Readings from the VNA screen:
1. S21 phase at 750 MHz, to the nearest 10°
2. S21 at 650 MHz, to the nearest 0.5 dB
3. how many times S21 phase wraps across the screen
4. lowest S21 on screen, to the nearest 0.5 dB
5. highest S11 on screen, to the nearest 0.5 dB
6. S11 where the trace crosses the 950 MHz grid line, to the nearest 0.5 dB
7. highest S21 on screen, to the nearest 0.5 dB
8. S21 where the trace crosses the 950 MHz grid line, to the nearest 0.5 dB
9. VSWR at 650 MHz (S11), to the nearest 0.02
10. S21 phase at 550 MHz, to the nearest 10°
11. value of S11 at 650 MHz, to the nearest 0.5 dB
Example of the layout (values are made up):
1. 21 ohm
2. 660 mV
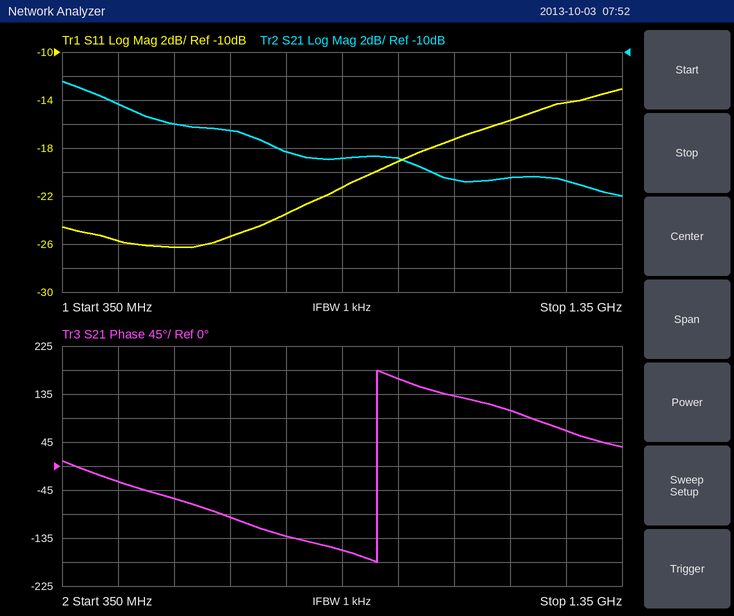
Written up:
1. -130°
2. -16.5 dB
3. 1
4. -22.0 dB
5. -13.0 dB
6. -19.0 dB
7. -12.5 dB
8. -19.0 dB
9. 1.12
10. -60°
11. -25.5 dB
